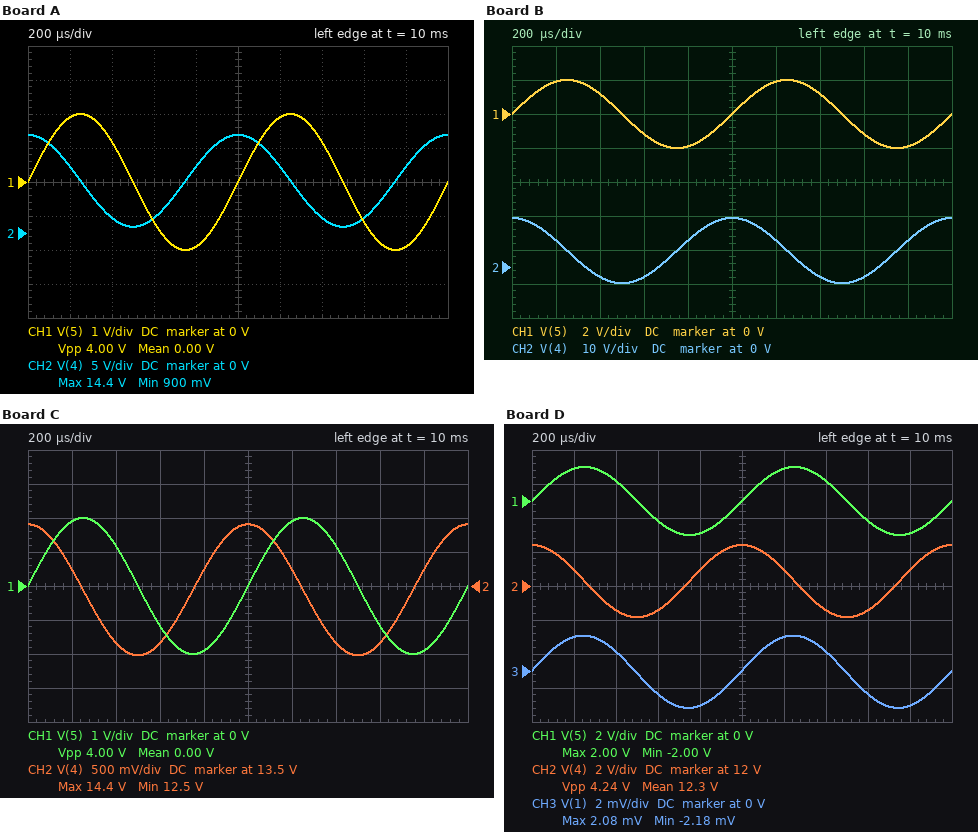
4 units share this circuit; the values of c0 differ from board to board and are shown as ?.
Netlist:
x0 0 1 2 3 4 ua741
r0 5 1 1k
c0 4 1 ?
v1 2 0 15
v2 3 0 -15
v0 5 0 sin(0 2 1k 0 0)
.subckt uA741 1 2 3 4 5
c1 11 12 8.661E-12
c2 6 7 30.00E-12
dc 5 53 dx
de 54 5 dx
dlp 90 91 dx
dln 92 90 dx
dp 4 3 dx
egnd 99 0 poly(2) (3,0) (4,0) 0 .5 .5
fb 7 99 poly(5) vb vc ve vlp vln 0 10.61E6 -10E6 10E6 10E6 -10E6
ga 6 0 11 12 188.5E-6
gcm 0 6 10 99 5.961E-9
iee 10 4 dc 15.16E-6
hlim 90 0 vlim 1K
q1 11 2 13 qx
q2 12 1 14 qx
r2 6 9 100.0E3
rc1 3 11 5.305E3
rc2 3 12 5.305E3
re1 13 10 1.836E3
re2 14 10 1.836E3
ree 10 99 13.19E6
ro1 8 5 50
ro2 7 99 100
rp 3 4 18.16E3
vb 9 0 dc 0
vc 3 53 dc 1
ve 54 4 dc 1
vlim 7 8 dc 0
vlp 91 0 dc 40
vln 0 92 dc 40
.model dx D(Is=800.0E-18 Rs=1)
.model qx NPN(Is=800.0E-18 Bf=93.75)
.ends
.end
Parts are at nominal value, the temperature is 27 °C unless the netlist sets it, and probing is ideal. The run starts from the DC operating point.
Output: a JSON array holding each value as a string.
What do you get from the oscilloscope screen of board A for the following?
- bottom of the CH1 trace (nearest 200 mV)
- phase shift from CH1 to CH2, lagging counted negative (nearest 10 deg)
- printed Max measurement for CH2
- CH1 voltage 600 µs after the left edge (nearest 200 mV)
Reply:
["-2.0 V", "90 deg", "14.4 V", "-1.2 V"]
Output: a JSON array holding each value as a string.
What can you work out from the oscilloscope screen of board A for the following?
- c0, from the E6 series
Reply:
["47 nF"]
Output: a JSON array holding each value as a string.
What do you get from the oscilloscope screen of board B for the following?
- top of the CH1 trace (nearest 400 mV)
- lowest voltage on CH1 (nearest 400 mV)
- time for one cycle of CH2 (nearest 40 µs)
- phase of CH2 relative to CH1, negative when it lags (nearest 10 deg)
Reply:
["2.0 V", "-2.0 V", "1.00 ms", "90 deg"]
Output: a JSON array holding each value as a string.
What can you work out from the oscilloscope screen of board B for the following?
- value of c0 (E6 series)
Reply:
["33 nF"]
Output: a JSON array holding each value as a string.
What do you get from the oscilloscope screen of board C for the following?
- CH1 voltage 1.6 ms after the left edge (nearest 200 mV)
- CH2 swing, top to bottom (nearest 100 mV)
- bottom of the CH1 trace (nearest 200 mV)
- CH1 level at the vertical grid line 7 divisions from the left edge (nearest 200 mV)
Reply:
["-1.2 V", "1.9 V", "-2.0 V", "1.2 V"]
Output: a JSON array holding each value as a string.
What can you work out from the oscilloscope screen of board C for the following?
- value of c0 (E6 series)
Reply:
["330 nF"]
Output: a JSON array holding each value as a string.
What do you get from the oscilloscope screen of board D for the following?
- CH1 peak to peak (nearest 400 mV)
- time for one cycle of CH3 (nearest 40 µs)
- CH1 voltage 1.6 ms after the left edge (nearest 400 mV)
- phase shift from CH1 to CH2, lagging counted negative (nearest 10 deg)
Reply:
["4.0 V", "1.00 ms", "-1.2 V", "90 deg"]
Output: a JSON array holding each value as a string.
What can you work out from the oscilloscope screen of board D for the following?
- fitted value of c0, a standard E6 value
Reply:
["150 nF"]
